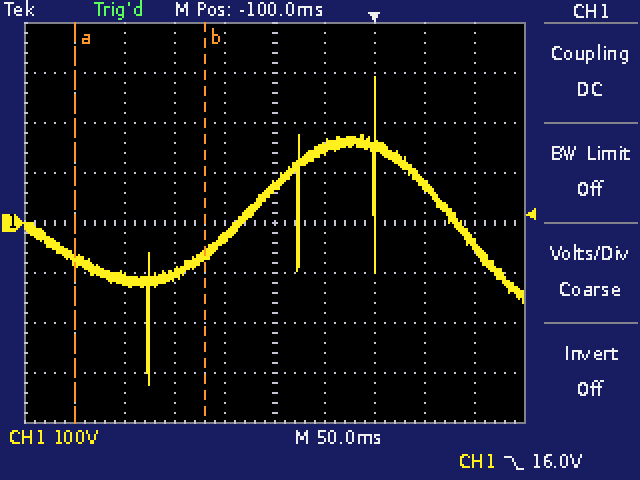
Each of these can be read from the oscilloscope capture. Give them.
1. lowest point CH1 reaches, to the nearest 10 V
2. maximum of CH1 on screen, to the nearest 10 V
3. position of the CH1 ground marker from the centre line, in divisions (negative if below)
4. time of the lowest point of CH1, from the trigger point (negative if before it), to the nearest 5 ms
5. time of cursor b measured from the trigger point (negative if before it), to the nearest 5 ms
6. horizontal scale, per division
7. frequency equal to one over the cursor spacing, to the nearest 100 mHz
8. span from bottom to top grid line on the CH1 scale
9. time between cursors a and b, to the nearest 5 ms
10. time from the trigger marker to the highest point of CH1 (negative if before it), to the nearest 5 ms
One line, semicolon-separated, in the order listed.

-320 V; 290 V; 0.0 div; -225 ms; -170 ms; 50 ms; 7.7 Hz; 800 V; 130 ms; 0 ms
